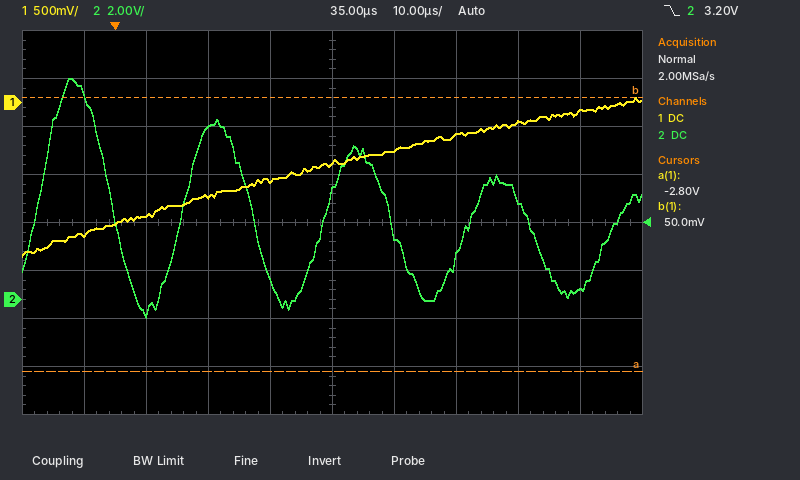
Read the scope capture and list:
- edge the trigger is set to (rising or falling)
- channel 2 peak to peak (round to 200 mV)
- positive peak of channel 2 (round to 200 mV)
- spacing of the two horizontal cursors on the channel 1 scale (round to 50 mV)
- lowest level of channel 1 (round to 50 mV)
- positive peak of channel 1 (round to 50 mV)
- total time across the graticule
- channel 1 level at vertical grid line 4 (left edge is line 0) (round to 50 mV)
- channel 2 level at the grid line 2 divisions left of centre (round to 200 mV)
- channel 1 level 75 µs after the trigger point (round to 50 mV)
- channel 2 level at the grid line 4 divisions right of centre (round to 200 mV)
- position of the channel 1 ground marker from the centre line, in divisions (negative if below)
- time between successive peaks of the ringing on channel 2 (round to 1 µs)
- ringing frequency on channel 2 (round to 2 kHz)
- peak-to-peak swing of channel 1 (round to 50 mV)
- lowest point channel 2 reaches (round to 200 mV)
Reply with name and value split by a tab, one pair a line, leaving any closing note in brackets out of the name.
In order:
edge the trigger is set to	falling
channel 2 peak to peak	10.0 V
positive peak of channel 2	9.2 V
spacing of the two horizontal cursors on the channel 1 scale	2.85 V
lowest level of channel 1	-1.60 V
positive peak of channel 1	50 mV
total time across the graticule	100 µs
channel 1 level at vertical grid line 4 (left edge is line 0)	-800 mV
channel 2 level at the grid line 2 divisions left of centre	7.2 V
channel 1 level 75 µs after the trigger point	-100 mV
channel 2 level at the grid line 4 divisions right of centre	400 mV
position of the channel 1 ground marker from the centre line, in divisions	+2.5 div
time between successive peaks of the ringing on channel 2	23 µs
ringing frequency on channel 2	44 kHz
peak-to-peak swing of channel 1	1.65 V
lowest point channel 2 reaches	-800 mV
